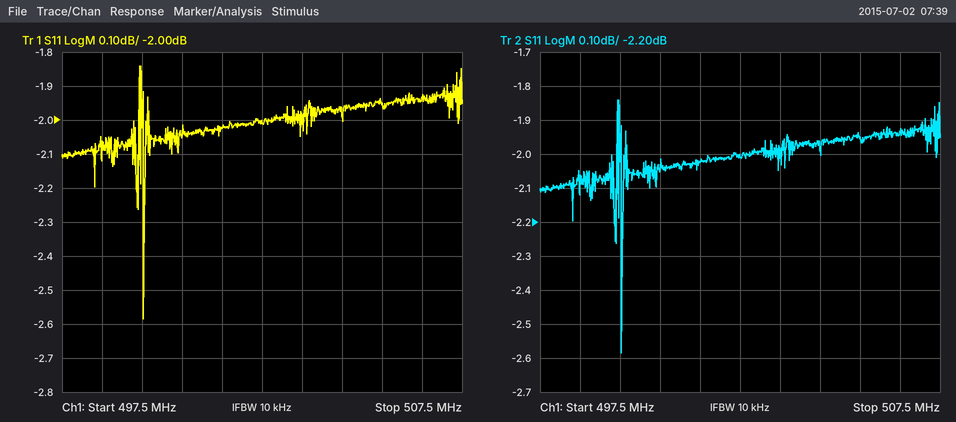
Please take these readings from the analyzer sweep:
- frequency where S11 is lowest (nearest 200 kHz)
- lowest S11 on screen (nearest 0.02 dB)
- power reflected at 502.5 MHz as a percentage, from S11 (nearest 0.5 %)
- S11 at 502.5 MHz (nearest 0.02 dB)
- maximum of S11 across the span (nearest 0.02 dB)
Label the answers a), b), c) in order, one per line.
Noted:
a) 499.6 MHz
b) -2.58 dB
c) 63.0 %
d) -2.00 dB
e) -1.84 dB
